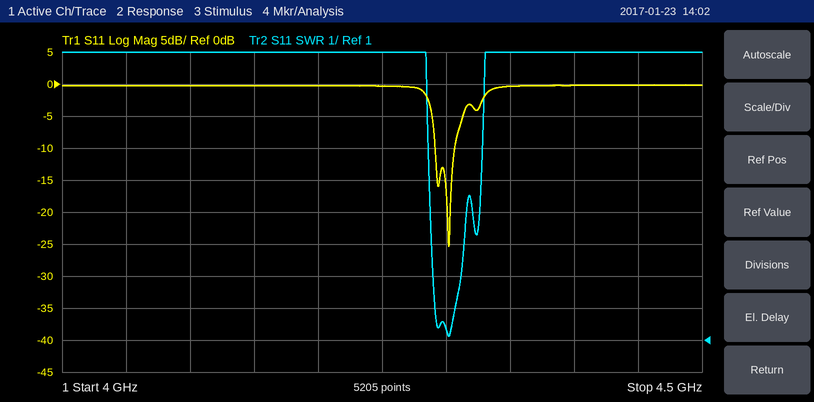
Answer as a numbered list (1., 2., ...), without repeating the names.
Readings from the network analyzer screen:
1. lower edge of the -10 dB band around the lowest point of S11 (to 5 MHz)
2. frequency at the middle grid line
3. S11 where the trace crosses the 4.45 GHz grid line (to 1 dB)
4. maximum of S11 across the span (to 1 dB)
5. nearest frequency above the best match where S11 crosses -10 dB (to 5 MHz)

1. 4.290 GHz
2. 4.25 GHz
3. 0 dB
4. 0 dB
5. 4.305 GHz
